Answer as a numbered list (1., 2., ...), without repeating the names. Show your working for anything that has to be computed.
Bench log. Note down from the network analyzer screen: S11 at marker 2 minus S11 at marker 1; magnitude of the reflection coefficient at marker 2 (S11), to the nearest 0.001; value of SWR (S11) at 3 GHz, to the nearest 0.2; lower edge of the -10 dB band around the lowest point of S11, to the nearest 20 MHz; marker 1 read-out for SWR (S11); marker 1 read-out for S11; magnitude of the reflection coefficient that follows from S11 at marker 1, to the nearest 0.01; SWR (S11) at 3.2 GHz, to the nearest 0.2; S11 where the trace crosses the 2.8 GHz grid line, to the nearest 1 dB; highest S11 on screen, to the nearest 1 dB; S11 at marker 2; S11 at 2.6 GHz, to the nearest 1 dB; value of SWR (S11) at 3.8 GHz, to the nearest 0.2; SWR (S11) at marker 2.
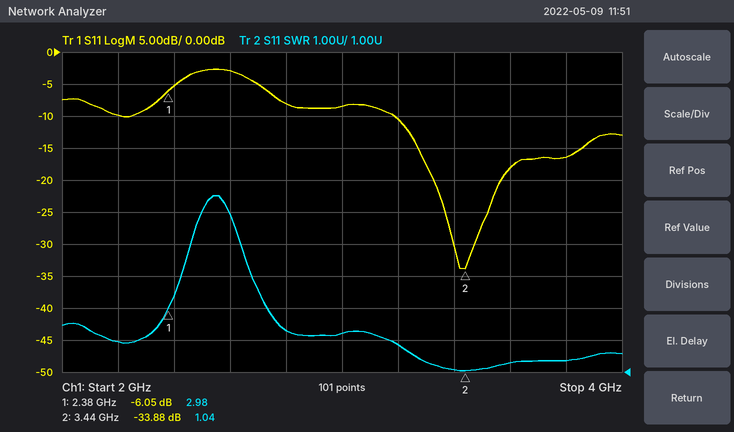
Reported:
1. -33.88 − (-6.05) = -27.83 dB
2. 10^(-33.88/20) ≈ 0.020
3. 2.2
4. 3.18 GHz
5. 2.98
6. -6.05 dB
7. 10^(-6.05/20) ≈ 0.50
8. 1.8
9. -8 dB
10. -3 dB
11. -33.88 dB
12. -3 dB
13. 1.4
14. 1.04
